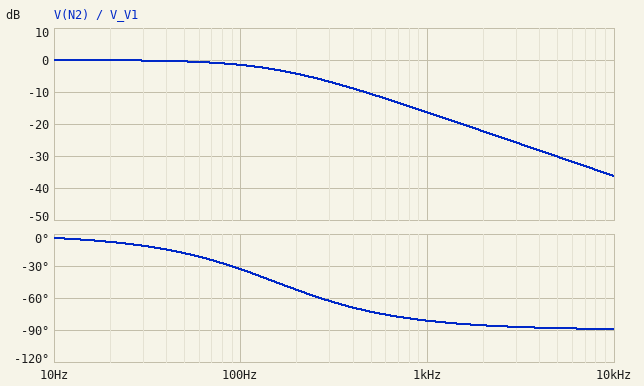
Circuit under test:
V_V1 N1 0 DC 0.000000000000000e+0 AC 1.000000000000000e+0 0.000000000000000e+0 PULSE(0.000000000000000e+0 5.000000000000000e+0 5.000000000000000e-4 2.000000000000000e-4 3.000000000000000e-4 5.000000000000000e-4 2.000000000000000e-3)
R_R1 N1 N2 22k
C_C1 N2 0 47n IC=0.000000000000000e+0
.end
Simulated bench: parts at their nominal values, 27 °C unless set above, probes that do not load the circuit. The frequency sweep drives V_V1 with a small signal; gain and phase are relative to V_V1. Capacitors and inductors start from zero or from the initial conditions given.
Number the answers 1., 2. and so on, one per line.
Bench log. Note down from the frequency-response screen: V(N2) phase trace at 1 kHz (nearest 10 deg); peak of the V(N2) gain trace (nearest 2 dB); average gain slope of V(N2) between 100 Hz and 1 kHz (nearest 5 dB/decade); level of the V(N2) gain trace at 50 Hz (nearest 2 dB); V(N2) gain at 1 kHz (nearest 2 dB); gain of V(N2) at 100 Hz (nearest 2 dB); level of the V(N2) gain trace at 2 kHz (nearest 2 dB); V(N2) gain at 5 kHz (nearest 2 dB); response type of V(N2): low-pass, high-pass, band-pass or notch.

1. -80 deg
2. 0 dB
3. -15 dB/decade
4. 0 dB
5. -16 dB
6. -2 dB
7. -22 dB
8. -30 dB
9. low-pass
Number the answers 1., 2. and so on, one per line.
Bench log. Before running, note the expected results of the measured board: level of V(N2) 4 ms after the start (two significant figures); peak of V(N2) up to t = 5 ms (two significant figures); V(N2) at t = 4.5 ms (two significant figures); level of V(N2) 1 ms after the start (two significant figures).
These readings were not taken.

1. 1.6 V
2. 2.8 V
3. 980 mV
4. 1.6 V
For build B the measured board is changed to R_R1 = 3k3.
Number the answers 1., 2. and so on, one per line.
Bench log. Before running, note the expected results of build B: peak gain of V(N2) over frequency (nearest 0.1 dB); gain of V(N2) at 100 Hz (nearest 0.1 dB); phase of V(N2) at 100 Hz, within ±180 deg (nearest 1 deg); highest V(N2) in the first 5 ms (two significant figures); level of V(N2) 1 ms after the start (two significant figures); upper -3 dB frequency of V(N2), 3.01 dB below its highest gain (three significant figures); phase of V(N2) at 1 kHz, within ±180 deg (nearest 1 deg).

1. 0 dB
2. 0 dB
3. -6 deg
4. 4.9 V
5. 4.6 V
6. 1.03 kHz
7. -44 deg
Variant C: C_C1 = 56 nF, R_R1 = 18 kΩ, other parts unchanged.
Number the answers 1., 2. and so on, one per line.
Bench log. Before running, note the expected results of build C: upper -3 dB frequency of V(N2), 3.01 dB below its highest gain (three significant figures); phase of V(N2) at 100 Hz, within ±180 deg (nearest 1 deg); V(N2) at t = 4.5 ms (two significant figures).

1. 158 Hz
2. -32 deg
3. 960 mV
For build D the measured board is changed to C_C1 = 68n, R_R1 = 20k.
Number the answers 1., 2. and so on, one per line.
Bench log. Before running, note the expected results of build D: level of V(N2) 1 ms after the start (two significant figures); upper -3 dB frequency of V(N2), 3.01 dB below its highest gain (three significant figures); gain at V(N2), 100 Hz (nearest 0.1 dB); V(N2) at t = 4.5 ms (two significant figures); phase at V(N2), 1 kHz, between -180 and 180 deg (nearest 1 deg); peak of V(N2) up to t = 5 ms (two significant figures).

1. 1.3 V
2. 117 Hz
3. -2.4 dB
4. 1.1 V
5. -83 deg
6. 2.5 V
